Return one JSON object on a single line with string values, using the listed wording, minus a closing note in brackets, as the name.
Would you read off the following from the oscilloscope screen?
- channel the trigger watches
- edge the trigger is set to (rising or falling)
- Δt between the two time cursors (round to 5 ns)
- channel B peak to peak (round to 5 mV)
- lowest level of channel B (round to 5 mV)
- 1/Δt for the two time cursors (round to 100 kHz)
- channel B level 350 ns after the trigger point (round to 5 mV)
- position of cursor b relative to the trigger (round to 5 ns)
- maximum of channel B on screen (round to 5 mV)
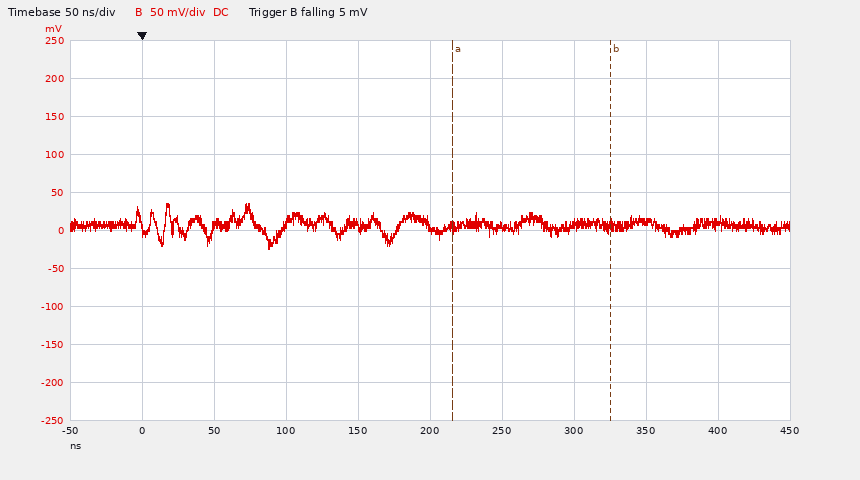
{"channel the trigger watches": "channel B", "edge the trigger is set to": "falling", "Δt between the two time cursors": "110 ns", "channel B peak to peak": "60 mV", "lowest level of channel B": "-25 mV", "1/Δt for the two time cursors": "9.1 MHz", "channel B level 350 ns after the trigger point": "10 mV", "position of cursor b relative to the trigger": "+325 ns", "maximum of channel B on screen": "35 mV"}
